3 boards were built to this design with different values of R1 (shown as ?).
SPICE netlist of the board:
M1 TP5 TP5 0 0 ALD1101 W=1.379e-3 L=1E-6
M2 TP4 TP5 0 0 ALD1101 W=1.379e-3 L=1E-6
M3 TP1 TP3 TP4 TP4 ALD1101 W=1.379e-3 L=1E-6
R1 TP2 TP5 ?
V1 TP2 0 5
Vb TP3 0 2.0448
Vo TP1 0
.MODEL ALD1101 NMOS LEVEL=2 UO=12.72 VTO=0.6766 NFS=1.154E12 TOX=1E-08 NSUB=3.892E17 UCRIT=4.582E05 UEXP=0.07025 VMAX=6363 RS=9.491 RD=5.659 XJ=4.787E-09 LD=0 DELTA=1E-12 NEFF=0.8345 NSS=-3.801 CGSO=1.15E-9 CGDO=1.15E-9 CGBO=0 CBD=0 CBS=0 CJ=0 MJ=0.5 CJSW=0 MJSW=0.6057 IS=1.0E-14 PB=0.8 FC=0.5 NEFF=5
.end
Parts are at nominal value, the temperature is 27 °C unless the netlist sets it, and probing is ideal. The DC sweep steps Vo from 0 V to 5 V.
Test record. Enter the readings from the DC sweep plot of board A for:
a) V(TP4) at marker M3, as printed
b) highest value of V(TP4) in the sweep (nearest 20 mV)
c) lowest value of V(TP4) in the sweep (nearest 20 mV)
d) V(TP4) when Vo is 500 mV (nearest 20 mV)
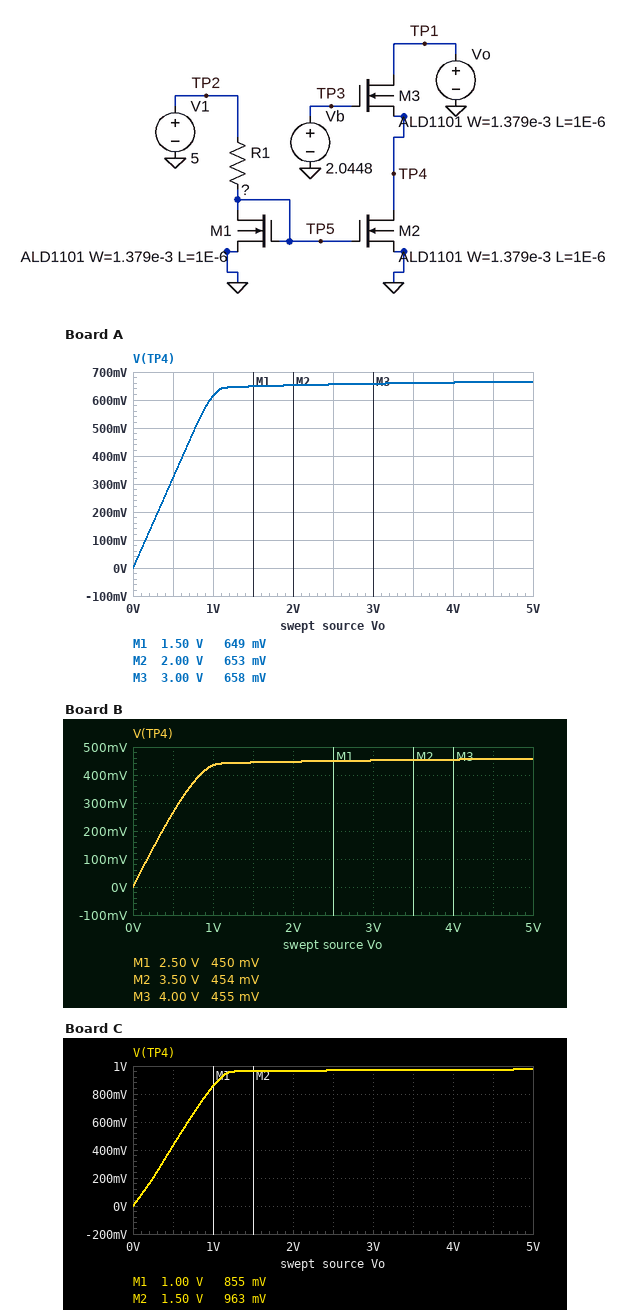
658 mV
660 mV
0 V
320 mV
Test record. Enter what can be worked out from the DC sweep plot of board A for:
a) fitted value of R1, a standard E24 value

3.3 kΩ
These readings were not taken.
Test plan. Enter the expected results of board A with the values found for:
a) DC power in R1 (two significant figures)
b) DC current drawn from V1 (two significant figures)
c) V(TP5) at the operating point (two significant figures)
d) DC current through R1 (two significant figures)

3.9 mW
1.1 mA
1.4 V
1.1 mA
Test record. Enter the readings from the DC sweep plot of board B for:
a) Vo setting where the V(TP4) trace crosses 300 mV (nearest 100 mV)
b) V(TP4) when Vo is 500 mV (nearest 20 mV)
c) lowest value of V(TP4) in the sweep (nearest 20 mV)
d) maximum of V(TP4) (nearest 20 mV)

600 mV
260 mV
0 V
460 mV
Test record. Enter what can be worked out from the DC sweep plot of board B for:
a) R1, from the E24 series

1.6 kΩ
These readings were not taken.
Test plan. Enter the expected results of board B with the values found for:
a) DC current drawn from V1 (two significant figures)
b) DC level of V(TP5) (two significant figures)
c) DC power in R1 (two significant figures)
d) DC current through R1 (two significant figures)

2.1 mA
1.7 V
6.9 mW
2.1 mA
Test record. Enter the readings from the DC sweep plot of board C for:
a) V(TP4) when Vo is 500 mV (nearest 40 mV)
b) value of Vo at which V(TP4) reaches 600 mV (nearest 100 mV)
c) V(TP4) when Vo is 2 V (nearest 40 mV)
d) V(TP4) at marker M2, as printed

440 mV
700 mV
960 mV
963 mV
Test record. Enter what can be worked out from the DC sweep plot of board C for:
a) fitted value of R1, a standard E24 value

11 kΩ
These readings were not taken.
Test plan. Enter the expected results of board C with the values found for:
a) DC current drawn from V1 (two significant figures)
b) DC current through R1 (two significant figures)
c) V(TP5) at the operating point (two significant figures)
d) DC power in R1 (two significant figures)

360 µA
360 µA
1.1 V
1.4 mW
